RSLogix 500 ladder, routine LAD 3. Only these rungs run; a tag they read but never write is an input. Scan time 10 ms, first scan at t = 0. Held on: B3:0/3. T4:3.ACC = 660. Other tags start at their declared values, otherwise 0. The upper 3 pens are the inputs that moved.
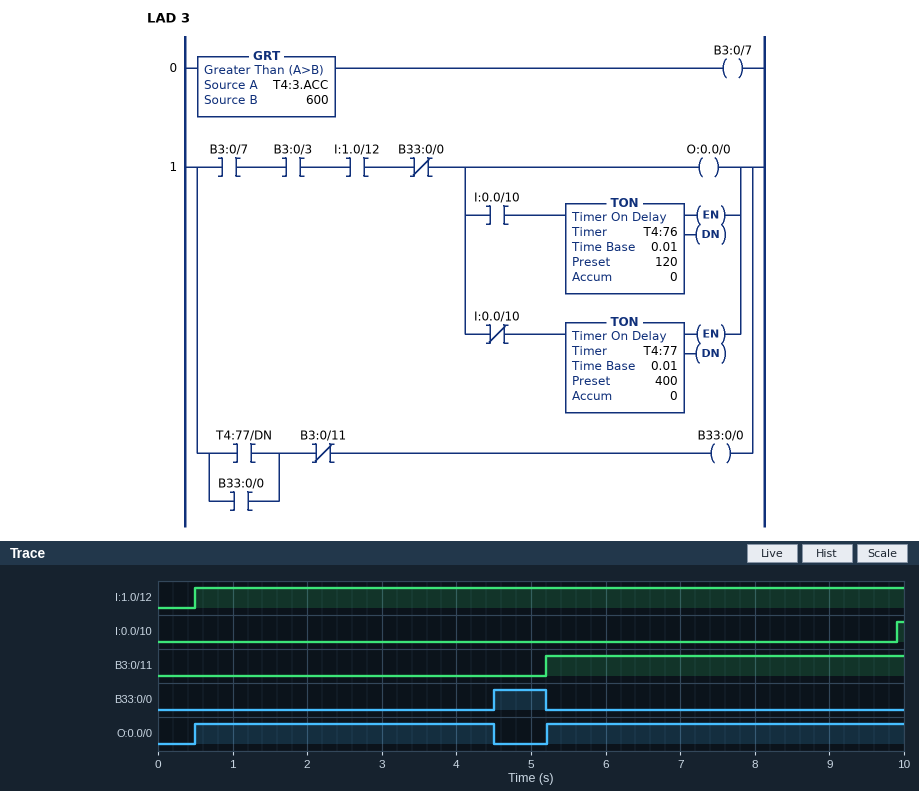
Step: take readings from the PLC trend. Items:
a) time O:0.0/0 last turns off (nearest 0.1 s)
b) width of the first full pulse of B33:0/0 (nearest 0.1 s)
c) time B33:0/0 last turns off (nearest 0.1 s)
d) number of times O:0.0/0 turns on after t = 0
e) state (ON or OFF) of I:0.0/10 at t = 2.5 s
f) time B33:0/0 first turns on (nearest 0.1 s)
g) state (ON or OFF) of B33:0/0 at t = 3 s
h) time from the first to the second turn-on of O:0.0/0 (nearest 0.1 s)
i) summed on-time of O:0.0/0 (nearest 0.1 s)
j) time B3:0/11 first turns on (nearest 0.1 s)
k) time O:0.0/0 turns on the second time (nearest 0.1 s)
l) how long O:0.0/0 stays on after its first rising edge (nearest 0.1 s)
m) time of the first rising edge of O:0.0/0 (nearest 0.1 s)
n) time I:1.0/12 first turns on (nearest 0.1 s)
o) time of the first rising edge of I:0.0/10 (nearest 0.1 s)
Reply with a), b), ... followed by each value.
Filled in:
a) 4.5 s
b) 0.7 s
c) 5.2 s
d) 2
e) OFF
f) 4.5 s
g) OFF
h) 4.7 s
i) 8.8 s
j) 5.2 s
k) 5.2 s
l) 4.0 s
m) 0.5 s
n) 0.5 s
o) 9.9 s
